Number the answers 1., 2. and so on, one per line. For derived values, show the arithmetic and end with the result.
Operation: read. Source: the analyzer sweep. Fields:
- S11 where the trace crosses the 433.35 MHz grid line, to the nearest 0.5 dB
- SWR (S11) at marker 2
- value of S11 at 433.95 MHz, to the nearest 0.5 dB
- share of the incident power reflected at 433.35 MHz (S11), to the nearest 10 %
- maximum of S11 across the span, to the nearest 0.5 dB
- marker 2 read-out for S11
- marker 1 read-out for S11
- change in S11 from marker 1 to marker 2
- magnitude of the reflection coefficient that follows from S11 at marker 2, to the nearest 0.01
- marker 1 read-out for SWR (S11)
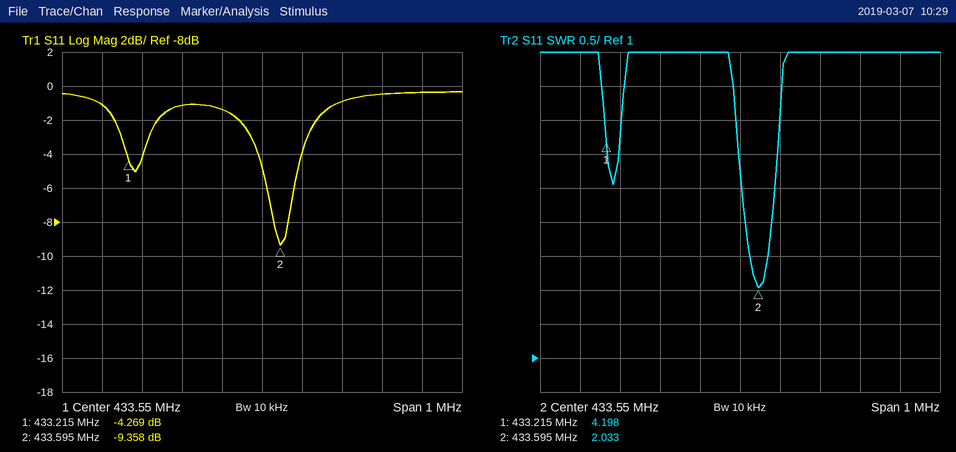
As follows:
1. -1.0 dB
2. 2.033
3. -0.5 dB
4. 10^(-1/10) ≈ 79.4 %, so 80 % to the nearest 10 %
5. -0.5 dB
6. -9.358 dB
7. -4.269 dB
8. -9.358 − (-4.269) = -5.089 dB
9. 10^(-9.358/20) ≈ 0.34
10. 4.198
